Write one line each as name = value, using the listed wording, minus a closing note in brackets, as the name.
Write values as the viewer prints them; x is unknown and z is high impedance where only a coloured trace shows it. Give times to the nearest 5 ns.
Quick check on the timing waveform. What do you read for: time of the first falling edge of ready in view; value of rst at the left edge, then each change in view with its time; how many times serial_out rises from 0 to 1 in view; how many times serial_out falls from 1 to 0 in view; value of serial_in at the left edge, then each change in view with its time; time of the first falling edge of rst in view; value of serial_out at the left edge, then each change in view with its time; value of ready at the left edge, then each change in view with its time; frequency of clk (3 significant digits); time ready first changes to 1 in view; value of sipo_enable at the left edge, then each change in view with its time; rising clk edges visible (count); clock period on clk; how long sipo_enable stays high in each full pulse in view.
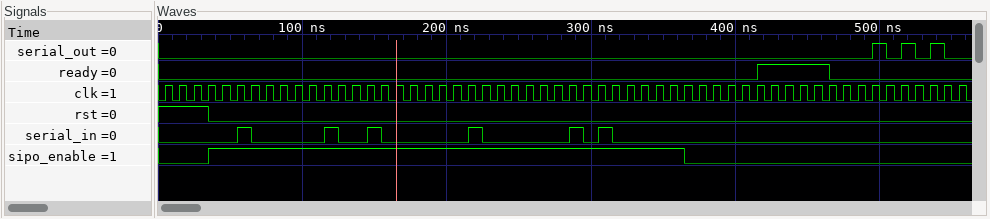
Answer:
time of the first falling edge of ready in view = 465 ns
value of rst at the left edge, then each change in view with its time = 1, 0 at 35 ns
how many times serial_out rises from 0 to 1 in view = 3
how many times serial_out falls from 1 to 0 in view = 3
value of serial_in at the left edge, then each change in view with its time = 0, 1 at 55 ns, 0 at 65 ns, 1 at 115 ns, 0 at 125 ns, 1 at 145 ns, 0 at 155 ns, 1 at 215 ns, 0 at 225 ns, 1 at 285 ns, 0 at 295 ns, 1 at 305 ns, 0 at 315 ns
time of the first falling edge of rst in view = 35 ns
value of serial_out at the left edge, then each change in view with its time = 0, 1 at 495 ns, 0 at 505 ns, 1 at 515 ns, 0 at 525 ns, 1 at 535 ns, 0 at 545 ns
value of ready at the left edge, then each change in view with its time = 0, 1 at 415 ns, 0 at 465 ns
frequency of clk = 100 MHz
time ready first changes to 1 in view = 415 ns
value of sipo_enable at the left edge, then each change in view with its time = 0, 1 at 35 ns, 0 at 365 ns
rising clk edges visible = 56
clock period on clk = 10 ns
how long sipo_enable stays high in each full pulse in view = 330 ns
